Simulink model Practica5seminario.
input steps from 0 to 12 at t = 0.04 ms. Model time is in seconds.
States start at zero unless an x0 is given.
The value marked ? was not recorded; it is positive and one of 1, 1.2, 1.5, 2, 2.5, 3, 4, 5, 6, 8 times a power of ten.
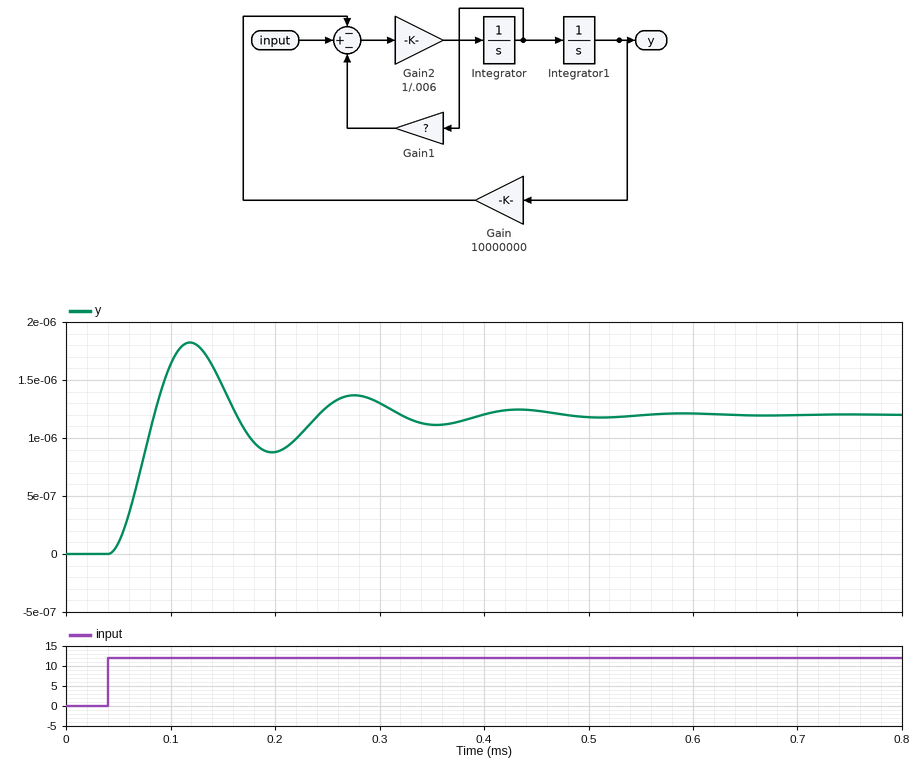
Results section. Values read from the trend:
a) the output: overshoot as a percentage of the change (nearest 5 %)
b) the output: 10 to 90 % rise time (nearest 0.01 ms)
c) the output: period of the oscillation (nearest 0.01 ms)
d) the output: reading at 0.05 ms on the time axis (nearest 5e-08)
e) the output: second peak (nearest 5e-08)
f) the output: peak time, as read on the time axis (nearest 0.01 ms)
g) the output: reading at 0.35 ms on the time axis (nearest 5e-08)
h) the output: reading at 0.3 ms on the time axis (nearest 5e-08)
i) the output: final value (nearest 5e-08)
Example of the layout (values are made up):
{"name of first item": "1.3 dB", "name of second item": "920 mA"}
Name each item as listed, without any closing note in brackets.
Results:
{"the output: overshoot as a percentage of the change": "50 %", "the output: 10 to 90 % rise time": "0.03 ms", "the output: period of the oscillation": "0.16 ms", "the output: reading at 0.05 ms on the time axis": "0.00000010", "the output: second peak": "0.00000135", "the output: peak time, as read on the time axis": "0.12 ms", "the output: reading at 0.35 ms on the time axis": "0.00000110", "the output: reading at 0.3 ms on the time axis": "0.00000130", "the output: final value": "0.00000120"}
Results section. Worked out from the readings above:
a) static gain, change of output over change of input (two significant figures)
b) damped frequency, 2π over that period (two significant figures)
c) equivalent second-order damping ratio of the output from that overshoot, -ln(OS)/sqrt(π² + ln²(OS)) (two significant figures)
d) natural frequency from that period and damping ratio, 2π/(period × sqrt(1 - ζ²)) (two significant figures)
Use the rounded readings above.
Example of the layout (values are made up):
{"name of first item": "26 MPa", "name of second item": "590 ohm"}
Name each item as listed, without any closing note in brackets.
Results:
{"static gain, change of output over change of input": "0.00000010", "damped frequency, 2π over that period": "39 rad/ms", "equivalent second-order damping ratio of the output from that overshoot, -ln(OS)/sqrt(π² + ln²(OS))": "0.22", "natural frequency from that period and damping ratio, 2π/(period × sqrt(1 - ζ²))": "40 rad/ms"}
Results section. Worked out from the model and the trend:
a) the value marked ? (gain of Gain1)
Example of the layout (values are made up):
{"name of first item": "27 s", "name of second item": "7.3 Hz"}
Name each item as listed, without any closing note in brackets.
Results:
{"the value marked ?": "100"}
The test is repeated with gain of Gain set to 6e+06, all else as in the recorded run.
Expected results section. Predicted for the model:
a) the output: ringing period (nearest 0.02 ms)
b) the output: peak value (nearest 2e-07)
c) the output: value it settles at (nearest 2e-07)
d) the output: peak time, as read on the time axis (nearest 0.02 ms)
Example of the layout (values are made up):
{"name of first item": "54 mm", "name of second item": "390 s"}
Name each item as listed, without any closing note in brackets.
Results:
{"the output: ringing period": "0.20 ms", "the output: peak value": "0.0000028", "the output: value it settles at": "0.0000020", "the output: peak time, as read on the time axis": "0.14 ms"}
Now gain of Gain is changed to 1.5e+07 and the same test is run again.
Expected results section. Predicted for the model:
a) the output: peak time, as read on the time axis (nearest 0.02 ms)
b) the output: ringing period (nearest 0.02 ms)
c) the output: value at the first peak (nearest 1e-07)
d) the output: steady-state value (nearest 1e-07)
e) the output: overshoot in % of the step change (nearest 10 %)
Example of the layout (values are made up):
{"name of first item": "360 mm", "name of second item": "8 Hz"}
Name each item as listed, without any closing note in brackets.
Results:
{"the output: peak time, as read on the time axis": "0.10 ms", "the output: ringing period": "0.12 ms", "the output: value at the first peak": "0.0000013", "the output: steady-state value": "0.0000008", "the output: overshoot in % of the step change": "60 %"}
